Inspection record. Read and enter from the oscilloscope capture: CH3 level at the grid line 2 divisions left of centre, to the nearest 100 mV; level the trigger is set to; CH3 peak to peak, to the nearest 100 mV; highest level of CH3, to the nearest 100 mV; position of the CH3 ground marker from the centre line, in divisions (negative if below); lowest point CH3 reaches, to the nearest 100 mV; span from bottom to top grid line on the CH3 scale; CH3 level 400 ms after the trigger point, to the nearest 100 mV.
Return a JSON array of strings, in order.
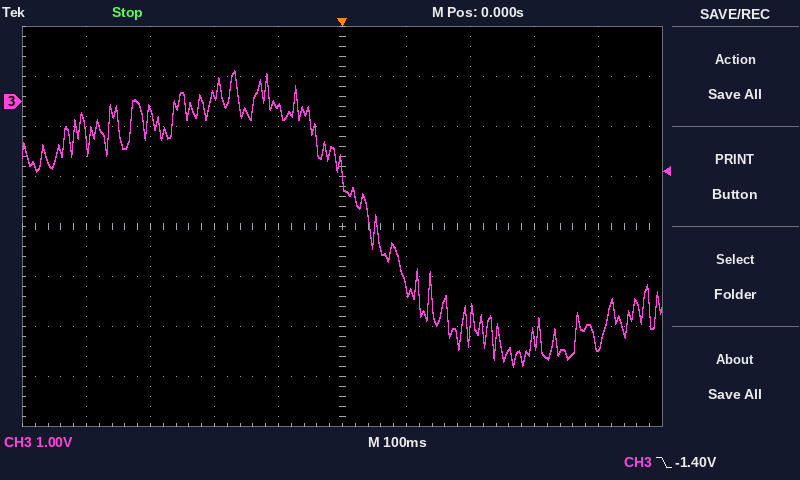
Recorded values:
["100 mV", "-1.40 V", "5.9 V", "600 mV", "+2.5 div", "-5.3 V", "8 V", "-4.9 V"]
